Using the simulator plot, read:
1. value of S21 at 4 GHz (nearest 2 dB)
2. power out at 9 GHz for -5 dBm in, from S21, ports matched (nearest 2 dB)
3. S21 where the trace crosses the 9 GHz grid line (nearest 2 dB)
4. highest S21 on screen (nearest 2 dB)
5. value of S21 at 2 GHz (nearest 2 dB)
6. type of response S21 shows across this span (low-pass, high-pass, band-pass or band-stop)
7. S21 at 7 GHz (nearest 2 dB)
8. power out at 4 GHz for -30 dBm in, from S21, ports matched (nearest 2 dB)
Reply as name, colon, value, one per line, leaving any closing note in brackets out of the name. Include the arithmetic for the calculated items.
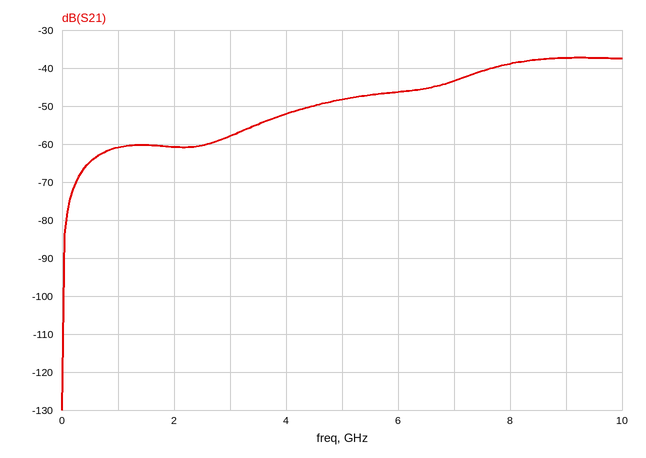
value of S21 at 4 GHz: -52 dB
power out at 9 GHz for -5 dBm in, from S21, ports matched: -5 dBm + (-38 dB) = -42 dBm
S21 where the trace crosses the 9 GHz grid line: -38 dB
highest S21 on screen: -38 dB
value of S21 at 2 GHz: -60 dB
type of response S21 shows across this span: high-pass
S21 at 7 GHz: -44 dB
power out at 4 GHz for -30 dBm in, from S21, ports matched: -30 dBm + (-52 dB) = -82 dBm
